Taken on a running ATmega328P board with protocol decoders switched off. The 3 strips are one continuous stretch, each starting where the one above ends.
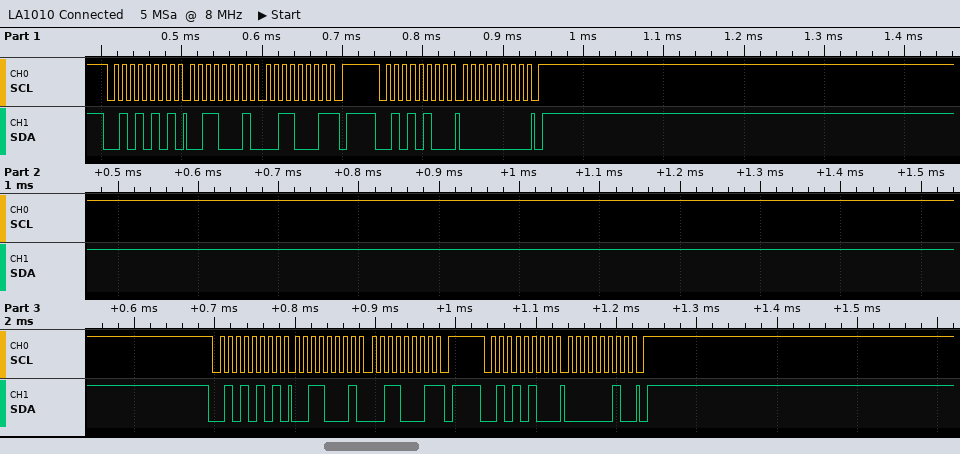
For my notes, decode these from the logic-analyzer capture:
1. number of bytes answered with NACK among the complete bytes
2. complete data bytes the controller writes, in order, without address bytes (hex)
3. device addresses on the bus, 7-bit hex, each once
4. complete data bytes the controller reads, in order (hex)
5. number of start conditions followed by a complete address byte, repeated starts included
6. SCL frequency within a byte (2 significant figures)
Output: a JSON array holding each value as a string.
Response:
["2", "00 02", "0x2A", "31 31 31 31", "4", "100 kHz"]
